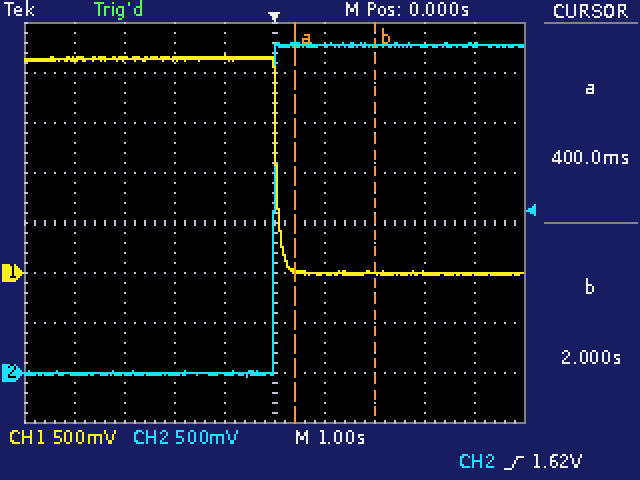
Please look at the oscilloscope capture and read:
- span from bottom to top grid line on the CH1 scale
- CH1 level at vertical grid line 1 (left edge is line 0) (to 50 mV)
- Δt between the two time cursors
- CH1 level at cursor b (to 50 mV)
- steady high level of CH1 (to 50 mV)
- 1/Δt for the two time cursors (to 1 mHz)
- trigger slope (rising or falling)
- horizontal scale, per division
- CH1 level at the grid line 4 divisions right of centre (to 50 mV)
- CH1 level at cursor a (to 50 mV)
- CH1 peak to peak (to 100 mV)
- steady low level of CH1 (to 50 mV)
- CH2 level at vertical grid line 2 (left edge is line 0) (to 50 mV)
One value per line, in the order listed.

4 V
2.15 V
1.6 s
0 mV
2.15 V
625 mHz
rising
1 s
0 mV
50 mV
2.20 V
0 mV
0 mV
